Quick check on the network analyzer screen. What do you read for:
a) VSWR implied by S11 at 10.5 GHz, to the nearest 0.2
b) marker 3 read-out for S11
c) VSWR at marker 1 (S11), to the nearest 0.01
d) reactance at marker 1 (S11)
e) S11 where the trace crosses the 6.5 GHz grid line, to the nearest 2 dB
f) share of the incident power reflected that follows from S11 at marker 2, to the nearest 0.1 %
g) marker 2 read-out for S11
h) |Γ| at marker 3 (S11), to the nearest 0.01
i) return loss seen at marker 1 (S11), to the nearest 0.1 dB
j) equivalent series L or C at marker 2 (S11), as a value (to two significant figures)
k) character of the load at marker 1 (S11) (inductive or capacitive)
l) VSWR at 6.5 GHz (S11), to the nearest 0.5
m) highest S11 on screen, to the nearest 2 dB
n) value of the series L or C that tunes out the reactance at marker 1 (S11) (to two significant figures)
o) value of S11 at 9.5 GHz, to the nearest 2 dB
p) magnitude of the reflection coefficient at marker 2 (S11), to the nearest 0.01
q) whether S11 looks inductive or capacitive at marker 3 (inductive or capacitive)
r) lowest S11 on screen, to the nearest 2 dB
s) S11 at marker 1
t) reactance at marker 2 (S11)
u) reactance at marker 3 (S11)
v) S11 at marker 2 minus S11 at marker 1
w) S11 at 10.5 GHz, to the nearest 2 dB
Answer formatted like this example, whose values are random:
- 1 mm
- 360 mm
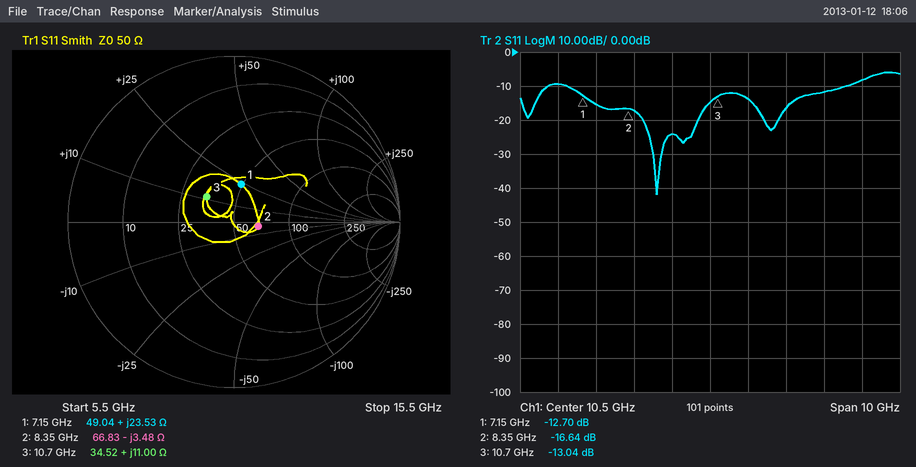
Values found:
- 1.4
- -13.04 dB
- 1.60
- +23.53 Ω
- -10 dB
- 2.2 %
- -16.64 dB
- 0.22
- 12.7 dB
- 5.5 pF
- inductive
- 2.0
- -6 dB
- 950 fF
- -24 dB
- 0.15
- inductive
- -42 dB
- -12.70 dB
- -3.48 Ω
- +11.00 Ω
- -3.94 dB
- -14 dB
